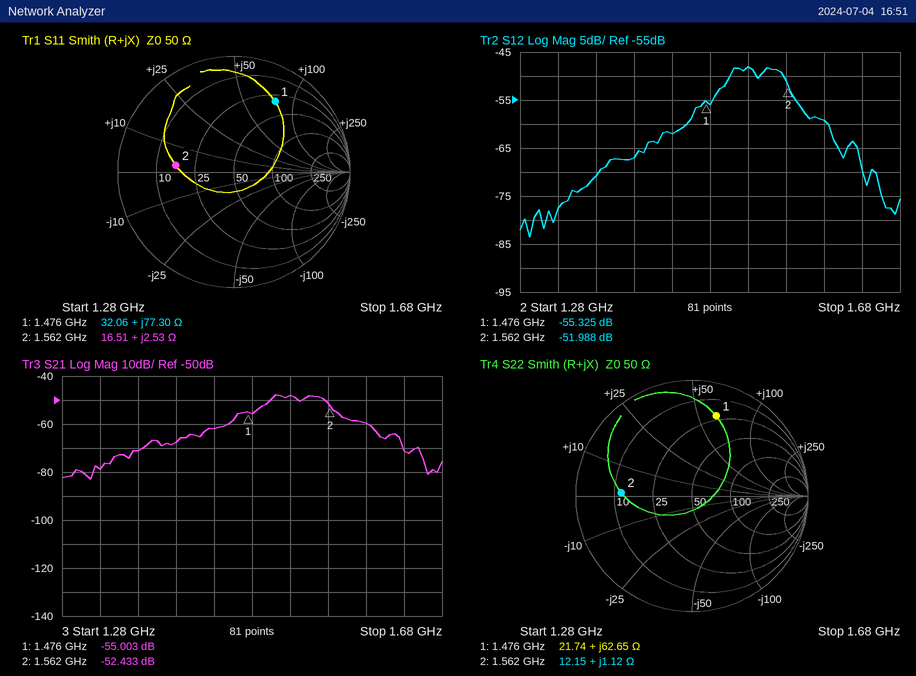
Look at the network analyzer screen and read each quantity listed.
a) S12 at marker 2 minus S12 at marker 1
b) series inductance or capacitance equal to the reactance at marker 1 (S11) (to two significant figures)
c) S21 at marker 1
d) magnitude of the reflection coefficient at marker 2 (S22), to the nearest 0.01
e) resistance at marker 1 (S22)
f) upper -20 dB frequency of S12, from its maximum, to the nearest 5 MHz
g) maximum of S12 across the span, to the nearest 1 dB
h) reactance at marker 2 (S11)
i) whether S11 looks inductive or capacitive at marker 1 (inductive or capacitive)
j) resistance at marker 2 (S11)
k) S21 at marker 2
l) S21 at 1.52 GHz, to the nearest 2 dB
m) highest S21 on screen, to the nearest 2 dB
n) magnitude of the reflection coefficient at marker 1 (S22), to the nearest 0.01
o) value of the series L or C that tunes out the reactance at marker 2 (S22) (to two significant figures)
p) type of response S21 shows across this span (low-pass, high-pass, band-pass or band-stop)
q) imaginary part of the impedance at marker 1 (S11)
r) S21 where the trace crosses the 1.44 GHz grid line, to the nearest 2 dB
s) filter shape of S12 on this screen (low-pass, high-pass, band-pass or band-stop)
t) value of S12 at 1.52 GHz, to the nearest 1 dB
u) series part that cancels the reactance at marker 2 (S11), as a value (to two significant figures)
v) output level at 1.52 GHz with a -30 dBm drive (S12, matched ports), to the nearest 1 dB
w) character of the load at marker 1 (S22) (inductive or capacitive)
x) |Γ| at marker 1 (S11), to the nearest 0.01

3.337 dB
8.3 nH
-55.003 dB
0.61
21.74 Ω
1.640 GHz
-48 dB
+2.53 Ω
inductive
16.51 Ω
-52.433 dB
-48 dB
-48 dB
0.72
91 pF
band-pass
+77.30 Ω
-62 dB
band-pass
-48 dB
40 pF
-78 dBm
inductive
0.70
